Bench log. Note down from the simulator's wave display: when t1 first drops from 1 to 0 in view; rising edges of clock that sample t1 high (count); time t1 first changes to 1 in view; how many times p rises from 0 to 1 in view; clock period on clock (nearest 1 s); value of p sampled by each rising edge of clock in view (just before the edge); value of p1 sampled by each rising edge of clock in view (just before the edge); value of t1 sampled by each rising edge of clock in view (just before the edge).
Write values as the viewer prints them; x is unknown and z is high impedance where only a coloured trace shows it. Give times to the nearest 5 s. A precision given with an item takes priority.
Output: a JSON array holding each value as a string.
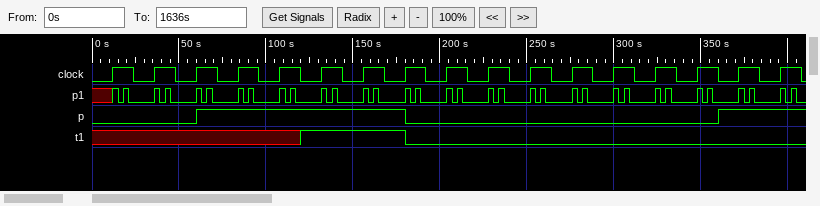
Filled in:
["180 s", "3", "120 s", "2", "24 s", "0 0 0 1 1 1 1 1 0 0 0 0 0 0 0 1 1", "x 0 0 0 0 0 0 0 0 0 0 0 0 0 0 0 0", "x x x x x 1 1 1 0 0 0 0 0 0 0 0 0"]
